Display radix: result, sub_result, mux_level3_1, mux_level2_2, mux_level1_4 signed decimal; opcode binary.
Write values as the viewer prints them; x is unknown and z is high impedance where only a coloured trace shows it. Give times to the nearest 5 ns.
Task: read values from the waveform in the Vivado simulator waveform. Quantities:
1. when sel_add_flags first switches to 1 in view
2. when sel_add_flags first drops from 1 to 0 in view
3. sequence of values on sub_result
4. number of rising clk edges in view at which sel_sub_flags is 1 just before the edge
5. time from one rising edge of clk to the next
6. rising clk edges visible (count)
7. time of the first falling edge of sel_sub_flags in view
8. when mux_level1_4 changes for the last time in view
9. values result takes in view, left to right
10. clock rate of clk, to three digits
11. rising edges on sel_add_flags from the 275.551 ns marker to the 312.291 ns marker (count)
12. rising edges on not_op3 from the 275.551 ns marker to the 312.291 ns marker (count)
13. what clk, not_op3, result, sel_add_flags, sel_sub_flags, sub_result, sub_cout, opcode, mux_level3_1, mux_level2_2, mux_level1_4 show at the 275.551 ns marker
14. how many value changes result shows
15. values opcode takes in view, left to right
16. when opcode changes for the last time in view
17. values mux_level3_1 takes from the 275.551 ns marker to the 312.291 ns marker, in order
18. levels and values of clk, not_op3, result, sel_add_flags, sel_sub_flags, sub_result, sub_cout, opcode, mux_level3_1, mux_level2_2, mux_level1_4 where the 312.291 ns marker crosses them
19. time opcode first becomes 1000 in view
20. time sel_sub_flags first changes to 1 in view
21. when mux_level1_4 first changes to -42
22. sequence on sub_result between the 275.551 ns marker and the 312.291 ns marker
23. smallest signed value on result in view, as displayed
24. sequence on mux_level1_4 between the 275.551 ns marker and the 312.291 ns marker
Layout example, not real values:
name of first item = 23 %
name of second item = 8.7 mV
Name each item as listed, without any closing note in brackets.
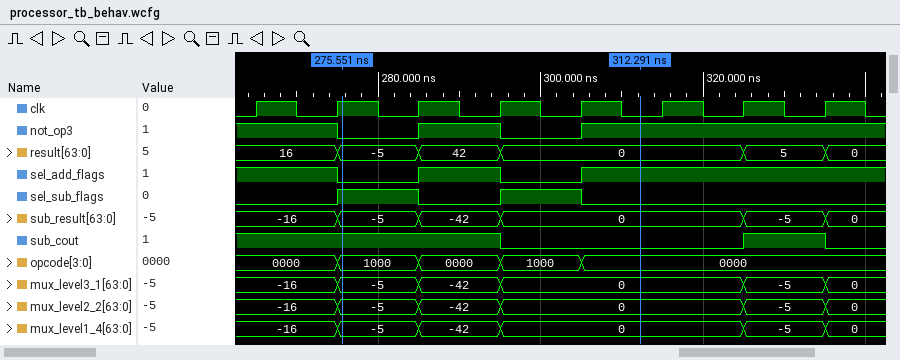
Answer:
when sel_add_flags first switches to 1 in view = 285 ns
when sel_add_flags first drops from 1 to 0 in view = 275 ns
sequence of values on sub_result = -16, -5, -42, 0, -5, 0
number of rising clk edges in view at which sel_sub_flags is 1 just before the edge = 2
time from one rising edge of clk to the next = 10 ns
rising clk edges visible = 8
time of the first falling edge of sel_sub_flags in view = 285 ns
when mux_level1_4 changes for the last time in view = 335 ns
values result takes in view, left to right = 16, -5, 42, 0, 5, 0
clock rate of clk, to three digits = 100 MHz
rising edges on sel_add_flags from the 275.551 ns marker to the 312.291 ns marker = 2
rising edges on not_op3 from the 275.551 ns marker to the 312.291 ns marker = 2
what clk, not_op3, result, sel_add_flags, sel_sub_flags, sub_result, sub_cout, opcode, mux_level3_1, mux_level2_2, mux_level1_4 show at the 275.551 ns marker = clk=1, not_op3=0, result=-5, sel_add_flags=0, sel_sub_flags=1, sub_result=-5, sub_cout=1, opcode=1000, mux_level3_1=-5, mux_level2_2=-5, mux_level1_4=-5
how many value changes result shows = 5
values opcode takes in view, left to right = 0000, 1000, 0000, 1000, 0000
when opcode changes for the last time in view = 305 ns
values mux_level3_1 takes from the 275.551 ns marker to the 312.291 ns marker, in order = -5, -42, 0
levels and values of clk, not_op3, result, sel_add_flags, sel_sub_flags, sub_result, sub_cout, opcode, mux_level3_1, mux_level2_2, mux_level1_4 where the 312.291 ns marker crosses them = clk=0, not_op3=1, result=0, sel_add_flags=1, sel_sub_flags=0, sub_result=0, sub_cout=0, opcode=0000, mux_level3_1=0, mux_level2_2=0, mux_level1_4=0
time opcode first becomes 1000 in view = 275 ns
time sel_sub_flags first changes to 1 in view = 275 ns
when mux_level1_4 first changes to -42 = 285 ns
sequence on sub_result between the 275.551 ns marker and the 312.291 ns marker = -5, -42, 0
smallest signed value on result in view, as displayed = -5
sequence on mux_level1_4 between the 275.551 ns marker and the 312.291 ns marker = -5, -42, 0
